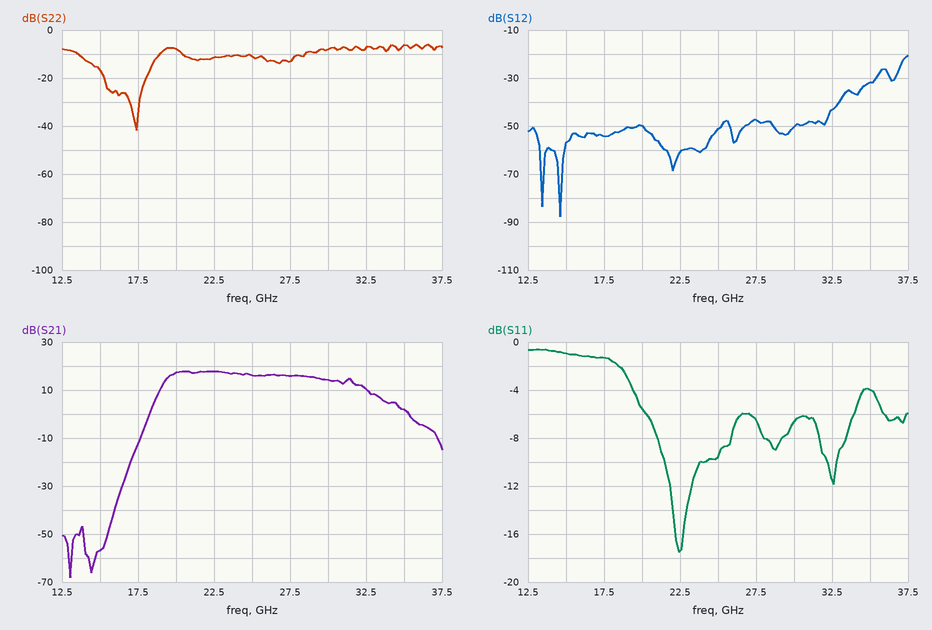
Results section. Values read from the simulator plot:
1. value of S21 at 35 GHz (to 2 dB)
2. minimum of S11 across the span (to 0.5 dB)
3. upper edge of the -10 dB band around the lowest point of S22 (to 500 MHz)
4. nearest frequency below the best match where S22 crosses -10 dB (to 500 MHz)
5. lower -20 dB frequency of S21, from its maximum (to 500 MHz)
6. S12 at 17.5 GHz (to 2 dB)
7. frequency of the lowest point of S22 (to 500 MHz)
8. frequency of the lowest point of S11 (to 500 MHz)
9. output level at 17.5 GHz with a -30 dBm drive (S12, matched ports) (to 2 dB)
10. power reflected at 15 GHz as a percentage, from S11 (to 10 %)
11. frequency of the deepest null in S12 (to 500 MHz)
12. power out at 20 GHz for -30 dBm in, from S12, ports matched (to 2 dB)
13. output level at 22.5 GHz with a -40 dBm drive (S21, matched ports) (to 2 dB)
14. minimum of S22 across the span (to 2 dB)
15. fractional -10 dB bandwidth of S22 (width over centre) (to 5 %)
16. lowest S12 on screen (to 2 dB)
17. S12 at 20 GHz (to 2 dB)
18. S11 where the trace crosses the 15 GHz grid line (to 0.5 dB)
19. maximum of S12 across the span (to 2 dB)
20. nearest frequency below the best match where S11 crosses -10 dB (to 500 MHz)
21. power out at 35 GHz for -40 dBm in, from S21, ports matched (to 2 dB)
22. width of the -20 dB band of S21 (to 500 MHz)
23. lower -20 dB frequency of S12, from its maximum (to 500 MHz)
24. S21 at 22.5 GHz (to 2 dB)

2 dB
-17.5 dB
19.0 GHz
13.5 GHz
18.0 GHz
-54 dB
17.5 GHz
22.5 GHz
-84 dBm
80 %
14.5 GHz
-80 dBm
-22 dBm
-42 dB
35 %
-88 dB
-50 dB
-1.0 dB
-20 dB
21.5 GHz
-38 dBm
17.5 GHz
33.0 GHz
18 dB
